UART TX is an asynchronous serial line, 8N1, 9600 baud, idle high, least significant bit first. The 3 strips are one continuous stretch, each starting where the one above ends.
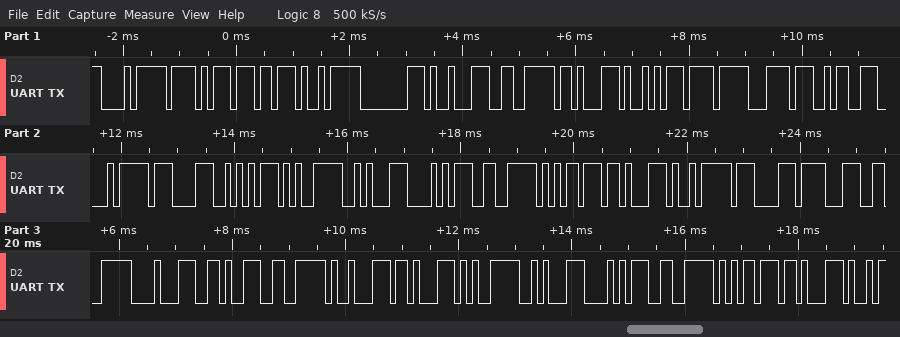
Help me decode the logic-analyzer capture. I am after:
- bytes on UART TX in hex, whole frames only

0xE8 0xAF 0xB7 0xE9 0x80 0x89 0xE6 0x8B 0xA9 0xEF 0xBC 0x9A 0xE8 0x87 0xAA 0xE5 0x8A 0xA8 0xE6 0xB5 0x8B 0xE9 0x87 0x8F 0xE6 0x88 0x96 0xE6 0x89 0x8B 0xE5 0x8A 0xA8 0xE6 0xB5 0x8B
